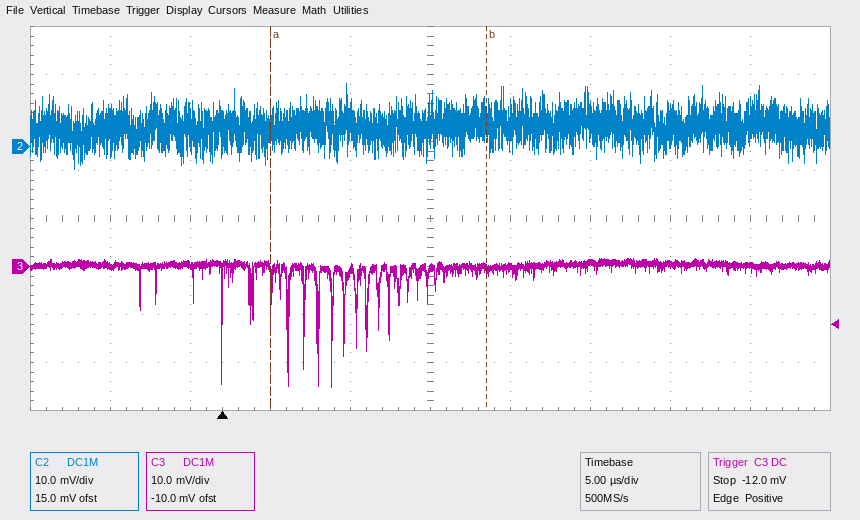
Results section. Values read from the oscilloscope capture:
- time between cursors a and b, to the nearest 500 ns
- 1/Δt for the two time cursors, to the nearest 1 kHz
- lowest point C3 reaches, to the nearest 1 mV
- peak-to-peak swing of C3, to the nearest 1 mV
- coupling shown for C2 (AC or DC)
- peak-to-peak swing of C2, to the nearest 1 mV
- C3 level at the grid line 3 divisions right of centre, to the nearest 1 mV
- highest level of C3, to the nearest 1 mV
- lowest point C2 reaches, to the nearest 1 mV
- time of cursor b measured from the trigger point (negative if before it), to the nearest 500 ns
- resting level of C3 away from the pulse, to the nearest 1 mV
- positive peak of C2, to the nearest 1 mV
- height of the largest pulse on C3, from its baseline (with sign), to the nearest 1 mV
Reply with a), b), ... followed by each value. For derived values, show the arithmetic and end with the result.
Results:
a) 13.5 µs
b) 1 / 13.5 µs ≈ 74 kHz
c) -25 mV
d) 2 mV − (-25 mV) = 27 mV
e) DC
f) 13 mV − (-5 mV) = 18 mV
g) 0 mV
h) 2 mV
i) -5 mV
j) +16.5 µs
k) 0 mV
l) 13 mV
m) -25 mV − (0 mV) = -25 mV
